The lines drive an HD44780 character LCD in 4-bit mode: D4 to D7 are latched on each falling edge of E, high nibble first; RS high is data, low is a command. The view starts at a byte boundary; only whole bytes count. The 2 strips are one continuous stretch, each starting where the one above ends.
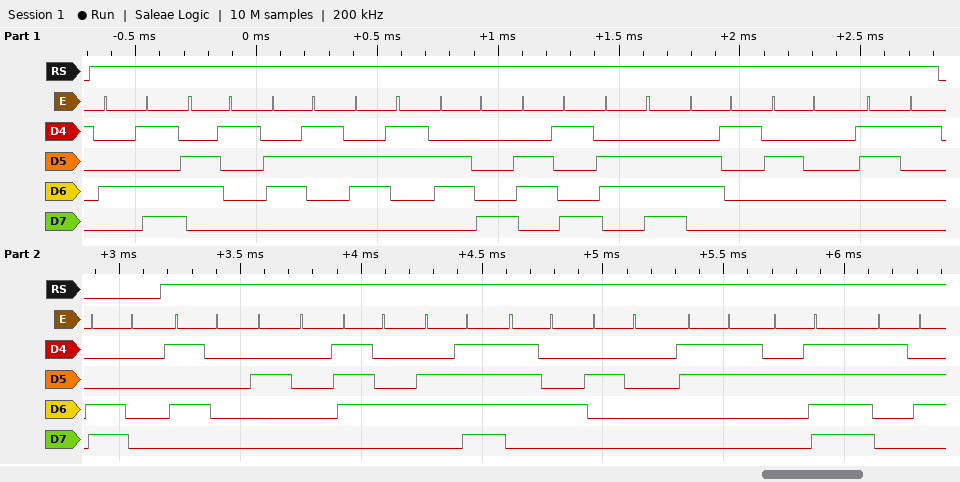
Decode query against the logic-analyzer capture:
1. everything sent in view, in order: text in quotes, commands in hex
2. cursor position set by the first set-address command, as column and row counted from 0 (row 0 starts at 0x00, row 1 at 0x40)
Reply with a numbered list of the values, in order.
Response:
1. "Macchina 1" 0xC0 "P tot 3/6"
2. column 0, row 1
